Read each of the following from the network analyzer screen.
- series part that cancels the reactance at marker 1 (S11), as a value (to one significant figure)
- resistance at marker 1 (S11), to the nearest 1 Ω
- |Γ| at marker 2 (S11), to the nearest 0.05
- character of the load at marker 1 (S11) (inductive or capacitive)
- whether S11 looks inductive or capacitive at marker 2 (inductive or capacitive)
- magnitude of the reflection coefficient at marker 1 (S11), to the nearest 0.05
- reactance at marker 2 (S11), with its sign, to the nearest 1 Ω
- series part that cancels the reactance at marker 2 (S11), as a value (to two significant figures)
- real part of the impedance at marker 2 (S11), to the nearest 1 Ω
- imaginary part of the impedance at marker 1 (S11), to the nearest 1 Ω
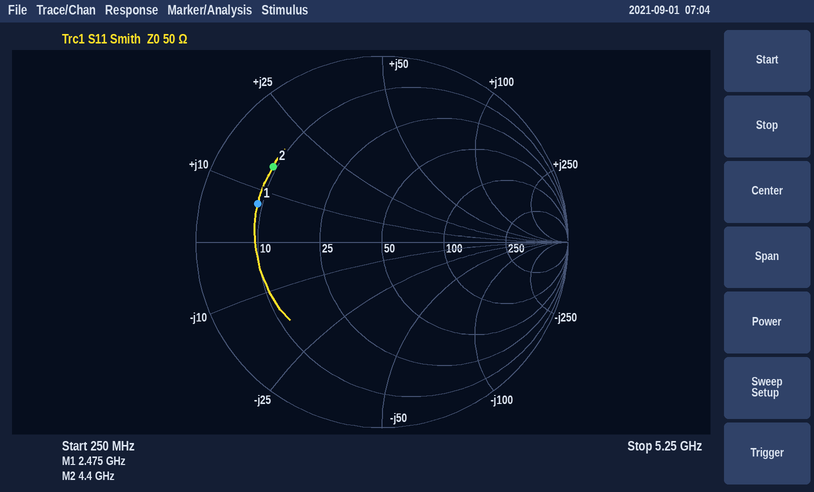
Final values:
9 pF
9 Ω
0.70
inductive
inductive
0.70
+15 Ω
2.4 pF
9 Ω
+7 Ω
